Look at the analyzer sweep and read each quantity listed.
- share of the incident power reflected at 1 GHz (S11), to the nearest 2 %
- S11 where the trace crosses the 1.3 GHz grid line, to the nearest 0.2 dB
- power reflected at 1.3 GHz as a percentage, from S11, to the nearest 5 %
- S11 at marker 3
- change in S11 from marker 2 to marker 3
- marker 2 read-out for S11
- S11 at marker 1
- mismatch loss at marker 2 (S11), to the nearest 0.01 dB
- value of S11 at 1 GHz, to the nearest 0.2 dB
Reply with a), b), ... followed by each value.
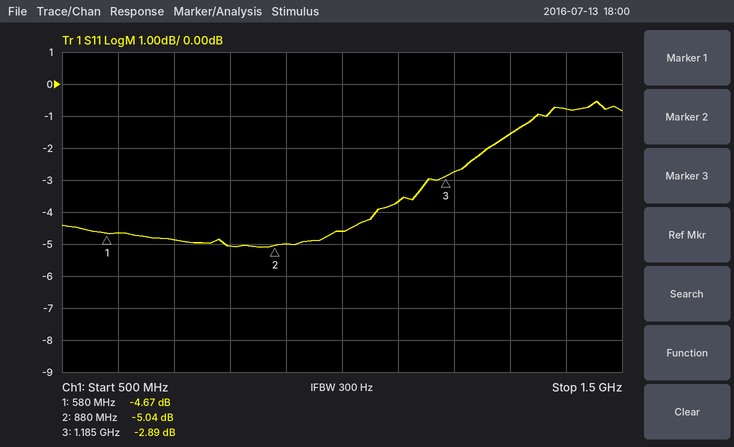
a) 34 %
b) -1.6 dB
c) 70 %
d) -2.89 dB
e) 2.15 dB
f) -5.04 dB
g) -4.67 dB
h) 1.63 dB
i) -4.6 dB
